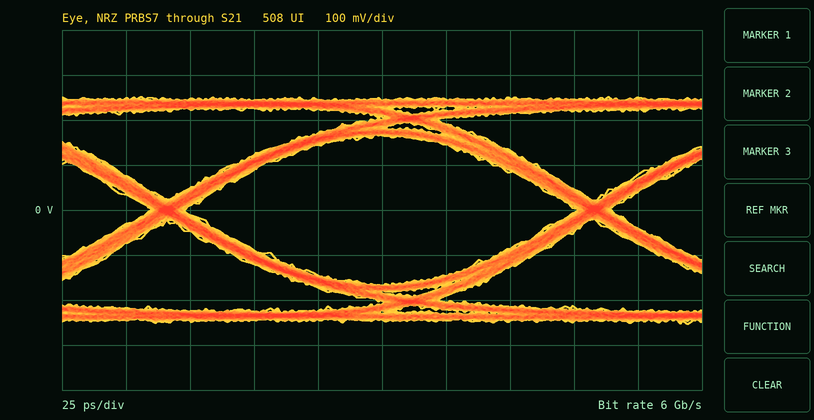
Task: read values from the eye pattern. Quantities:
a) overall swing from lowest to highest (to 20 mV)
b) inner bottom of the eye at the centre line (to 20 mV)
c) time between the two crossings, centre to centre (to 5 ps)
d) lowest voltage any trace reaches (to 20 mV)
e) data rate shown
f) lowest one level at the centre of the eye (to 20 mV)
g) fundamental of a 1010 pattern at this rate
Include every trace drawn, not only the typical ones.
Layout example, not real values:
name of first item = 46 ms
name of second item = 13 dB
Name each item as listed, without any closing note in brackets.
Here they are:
overall swing from lowest to highest = 500 mV
inner bottom of the eye at the centre line = -160 mV
time between the two crossings, centre to centre = 165 ps
lowest voltage any trace reaches = -260 mV
data rate shown = 6 Gb/s
lowest one level at the centre of the eye = 160 mV
fundamental of a 1010 pattern at this rate = 3 GHz
